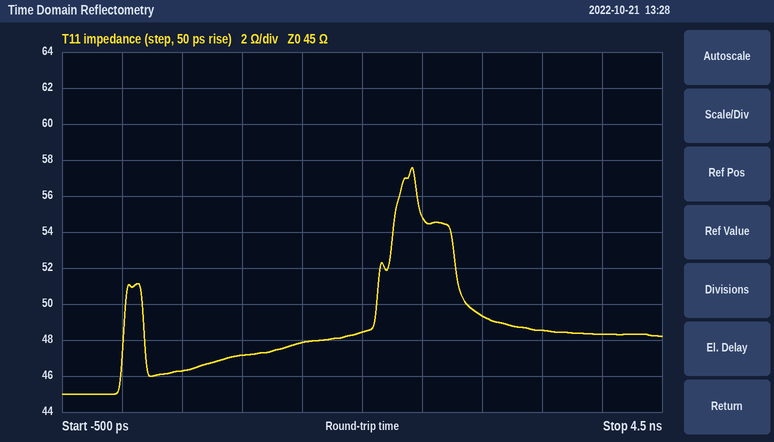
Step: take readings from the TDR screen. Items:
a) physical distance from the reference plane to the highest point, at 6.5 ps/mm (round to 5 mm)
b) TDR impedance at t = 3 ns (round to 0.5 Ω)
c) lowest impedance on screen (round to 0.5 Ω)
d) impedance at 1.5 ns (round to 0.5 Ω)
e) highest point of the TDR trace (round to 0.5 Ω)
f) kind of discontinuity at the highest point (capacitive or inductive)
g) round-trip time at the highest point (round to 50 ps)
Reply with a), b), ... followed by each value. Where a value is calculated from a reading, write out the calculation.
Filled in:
a) 2.40 ns / 2 / 6.5 ps/mm ≈ 185 mm
b) 49.5 Ω
c) 45.0 Ω
d) 48.0 Ω
e) 57.5 Ω
f) inductive
g) 2.40 ns
